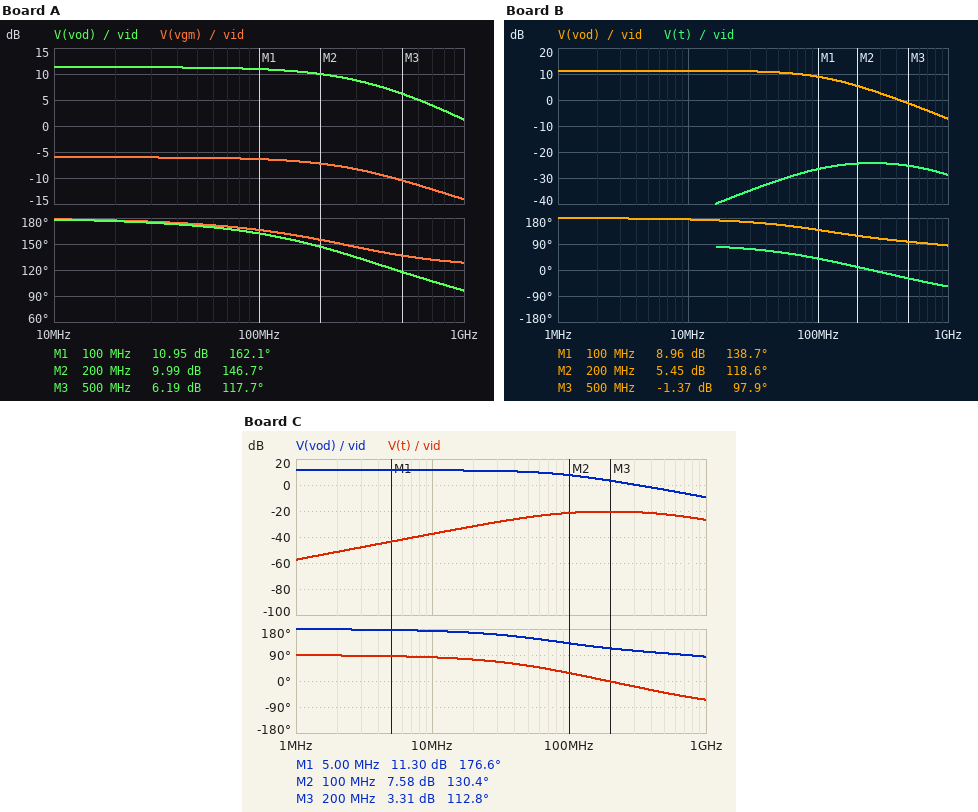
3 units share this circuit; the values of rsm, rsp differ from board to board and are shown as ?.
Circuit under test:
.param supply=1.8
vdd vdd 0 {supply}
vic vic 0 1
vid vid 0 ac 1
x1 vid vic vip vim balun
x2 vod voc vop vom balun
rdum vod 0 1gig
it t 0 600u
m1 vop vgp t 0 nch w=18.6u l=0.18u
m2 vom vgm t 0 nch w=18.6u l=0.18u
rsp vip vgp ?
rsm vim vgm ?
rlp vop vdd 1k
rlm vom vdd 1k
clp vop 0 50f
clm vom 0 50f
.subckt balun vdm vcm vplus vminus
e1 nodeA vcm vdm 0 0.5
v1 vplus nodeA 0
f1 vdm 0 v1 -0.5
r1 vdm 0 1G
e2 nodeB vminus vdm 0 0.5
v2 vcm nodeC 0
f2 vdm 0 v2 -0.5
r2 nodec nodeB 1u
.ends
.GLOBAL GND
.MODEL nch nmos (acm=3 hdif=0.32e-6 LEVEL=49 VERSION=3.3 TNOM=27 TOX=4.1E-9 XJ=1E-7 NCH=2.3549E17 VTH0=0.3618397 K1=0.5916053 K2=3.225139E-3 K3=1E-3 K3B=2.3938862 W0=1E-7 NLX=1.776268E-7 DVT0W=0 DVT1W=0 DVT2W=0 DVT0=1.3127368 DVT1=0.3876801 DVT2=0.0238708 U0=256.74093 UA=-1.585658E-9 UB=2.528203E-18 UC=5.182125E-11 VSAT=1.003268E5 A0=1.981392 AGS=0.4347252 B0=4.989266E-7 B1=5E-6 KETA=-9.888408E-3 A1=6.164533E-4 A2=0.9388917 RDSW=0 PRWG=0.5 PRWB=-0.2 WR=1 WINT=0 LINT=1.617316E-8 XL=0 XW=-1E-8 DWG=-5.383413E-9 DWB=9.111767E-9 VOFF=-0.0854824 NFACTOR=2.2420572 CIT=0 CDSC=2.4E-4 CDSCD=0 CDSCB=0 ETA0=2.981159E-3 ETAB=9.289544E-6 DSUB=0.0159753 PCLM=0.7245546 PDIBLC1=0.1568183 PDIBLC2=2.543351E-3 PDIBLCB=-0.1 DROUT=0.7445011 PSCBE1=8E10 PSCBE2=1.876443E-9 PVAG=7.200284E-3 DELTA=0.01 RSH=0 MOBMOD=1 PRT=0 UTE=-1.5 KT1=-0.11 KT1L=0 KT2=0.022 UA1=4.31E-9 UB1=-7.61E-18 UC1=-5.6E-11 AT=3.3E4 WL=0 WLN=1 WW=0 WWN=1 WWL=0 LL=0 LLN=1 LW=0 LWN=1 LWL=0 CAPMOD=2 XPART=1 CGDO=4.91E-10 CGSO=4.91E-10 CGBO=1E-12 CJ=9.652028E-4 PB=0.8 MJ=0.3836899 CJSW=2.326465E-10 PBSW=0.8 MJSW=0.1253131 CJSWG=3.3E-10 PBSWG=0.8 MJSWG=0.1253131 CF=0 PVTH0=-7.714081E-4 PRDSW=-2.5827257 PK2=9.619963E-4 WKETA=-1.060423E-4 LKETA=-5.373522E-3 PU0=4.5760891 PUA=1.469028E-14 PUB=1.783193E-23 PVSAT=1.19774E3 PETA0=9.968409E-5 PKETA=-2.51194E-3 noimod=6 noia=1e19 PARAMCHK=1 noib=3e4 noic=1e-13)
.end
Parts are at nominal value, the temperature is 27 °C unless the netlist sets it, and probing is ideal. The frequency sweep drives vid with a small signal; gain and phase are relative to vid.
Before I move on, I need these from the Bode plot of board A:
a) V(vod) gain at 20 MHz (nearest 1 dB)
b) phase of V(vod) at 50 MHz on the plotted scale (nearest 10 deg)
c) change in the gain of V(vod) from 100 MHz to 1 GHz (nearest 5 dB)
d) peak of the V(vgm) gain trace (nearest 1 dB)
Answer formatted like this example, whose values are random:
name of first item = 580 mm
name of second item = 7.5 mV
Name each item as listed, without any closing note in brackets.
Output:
V(vod) gain at 20 MHz = 11 dB
phase of V(vod) at 50 MHz on the plotted scale = 170 deg
change in the gain of V(vod) from 100 MHz to 1 GHz = -10 dB
peak of the V(vgm) gain trace = -6 dB
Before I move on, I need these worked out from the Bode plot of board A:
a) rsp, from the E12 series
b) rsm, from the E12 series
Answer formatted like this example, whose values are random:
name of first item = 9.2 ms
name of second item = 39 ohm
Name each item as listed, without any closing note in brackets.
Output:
rsp, from the E12 series = 6.8 kΩ
rsm, from the E12 series = 5.6 kΩ
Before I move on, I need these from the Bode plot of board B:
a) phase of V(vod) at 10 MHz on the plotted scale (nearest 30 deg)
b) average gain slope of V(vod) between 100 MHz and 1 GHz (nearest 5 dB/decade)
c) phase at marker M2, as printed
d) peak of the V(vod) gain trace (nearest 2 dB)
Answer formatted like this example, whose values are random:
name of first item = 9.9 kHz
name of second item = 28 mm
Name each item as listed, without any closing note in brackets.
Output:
phase of V(vod) at 10 MHz on the plotted scale = 180 deg
average gain slope of V(vod) between 100 MHz and 1 GHz = -15 dB/decade
phase at marker M2, as printed = 118.6 deg
peak of the V(vod) gain trace = 12 dB
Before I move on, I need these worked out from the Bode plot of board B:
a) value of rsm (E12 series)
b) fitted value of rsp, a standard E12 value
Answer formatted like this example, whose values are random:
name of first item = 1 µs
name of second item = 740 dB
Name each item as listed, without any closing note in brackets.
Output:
value of rsm = 22 kΩ
fitted value of rsp, a standard E12 value = 15 kΩ
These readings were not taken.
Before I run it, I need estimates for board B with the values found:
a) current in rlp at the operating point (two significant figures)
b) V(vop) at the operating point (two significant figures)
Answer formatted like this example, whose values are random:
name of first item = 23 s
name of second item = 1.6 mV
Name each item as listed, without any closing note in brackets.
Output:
current in rlp at the operating point = 300 µA
V(vop) at the operating point = 1.5 V
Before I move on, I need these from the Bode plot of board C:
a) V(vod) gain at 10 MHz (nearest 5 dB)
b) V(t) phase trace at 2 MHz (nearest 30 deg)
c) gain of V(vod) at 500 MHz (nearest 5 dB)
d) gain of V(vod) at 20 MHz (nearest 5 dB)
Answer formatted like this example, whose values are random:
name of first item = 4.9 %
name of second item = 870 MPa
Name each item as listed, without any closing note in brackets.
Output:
V(vod) gain at 10 MHz = 10 dB
V(t) phase trace at 2 MHz = 90 deg
gain of V(vod) at 500 MHz = -5 dB
gain of V(vod) at 20 MHz = 10 dB
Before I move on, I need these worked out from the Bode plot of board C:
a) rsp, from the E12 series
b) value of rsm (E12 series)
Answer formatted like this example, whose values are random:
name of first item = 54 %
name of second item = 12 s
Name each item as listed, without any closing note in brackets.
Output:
rsp, from the E12 series = 18 kΩ
value of rsm = 33 kΩ
